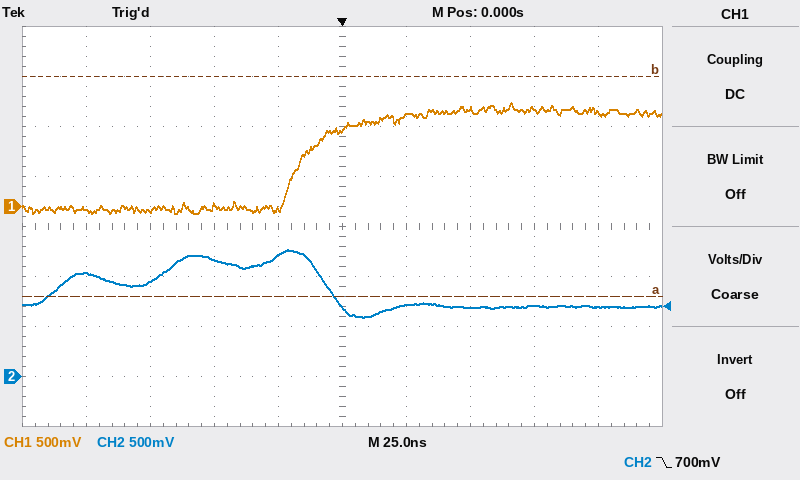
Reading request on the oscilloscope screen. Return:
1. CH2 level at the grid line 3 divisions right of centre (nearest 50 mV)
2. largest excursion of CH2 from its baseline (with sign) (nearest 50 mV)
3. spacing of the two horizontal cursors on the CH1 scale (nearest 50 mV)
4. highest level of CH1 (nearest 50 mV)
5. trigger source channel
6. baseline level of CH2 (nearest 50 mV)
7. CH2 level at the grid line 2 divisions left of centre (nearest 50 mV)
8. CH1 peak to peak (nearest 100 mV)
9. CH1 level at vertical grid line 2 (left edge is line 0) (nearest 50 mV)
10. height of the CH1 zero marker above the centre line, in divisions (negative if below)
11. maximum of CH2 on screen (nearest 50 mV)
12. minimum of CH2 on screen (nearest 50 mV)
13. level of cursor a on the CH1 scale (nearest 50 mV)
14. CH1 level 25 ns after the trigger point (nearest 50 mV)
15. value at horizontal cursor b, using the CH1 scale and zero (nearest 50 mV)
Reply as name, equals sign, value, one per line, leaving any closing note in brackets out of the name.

CH2 level at the grid line 3 divisions right of centre = 700 mV
largest excursion of CH2 from its baseline (with sign) = +550 mV
spacing of the two horizontal cursors on the CH1 scale = 2.20 V
highest level of CH1 = 1.05 V
trigger source channel = CH2
baseline level of CH2 = 700 mV
CH2 level at the grid line 2 divisions left of centre = 1.15 V
CH1 peak to peak = 1.10 V
CH1 level at vertical grid line 2 (left edge is line 0) = -50 mV
height of the CH1 zero marker above the centre line, in divisions = +0.4 div
maximum of CH2 on screen = 1.25 V
minimum of CH2 on screen = 600 mV
level of cursor a on the CH1 scale = -900 mV
CH1 level 25 ns after the trigger point = 900 mV
value at horizontal cursor b, using the CH1 scale and zero = 1.30 V
